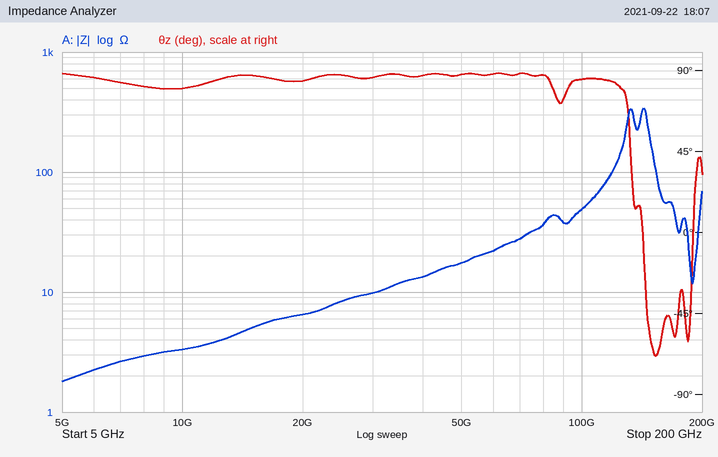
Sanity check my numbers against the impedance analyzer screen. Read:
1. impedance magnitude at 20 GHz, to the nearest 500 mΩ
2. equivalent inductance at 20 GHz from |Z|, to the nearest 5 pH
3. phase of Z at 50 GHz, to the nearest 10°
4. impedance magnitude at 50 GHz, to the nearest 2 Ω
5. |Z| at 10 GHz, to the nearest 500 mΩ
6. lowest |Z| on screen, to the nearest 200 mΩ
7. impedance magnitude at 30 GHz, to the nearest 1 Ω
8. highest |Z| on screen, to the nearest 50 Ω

6.5 Ω
50 pH
90°
18 Ω
3.5 Ω
1.8 Ω
10 Ω
350 Ω
